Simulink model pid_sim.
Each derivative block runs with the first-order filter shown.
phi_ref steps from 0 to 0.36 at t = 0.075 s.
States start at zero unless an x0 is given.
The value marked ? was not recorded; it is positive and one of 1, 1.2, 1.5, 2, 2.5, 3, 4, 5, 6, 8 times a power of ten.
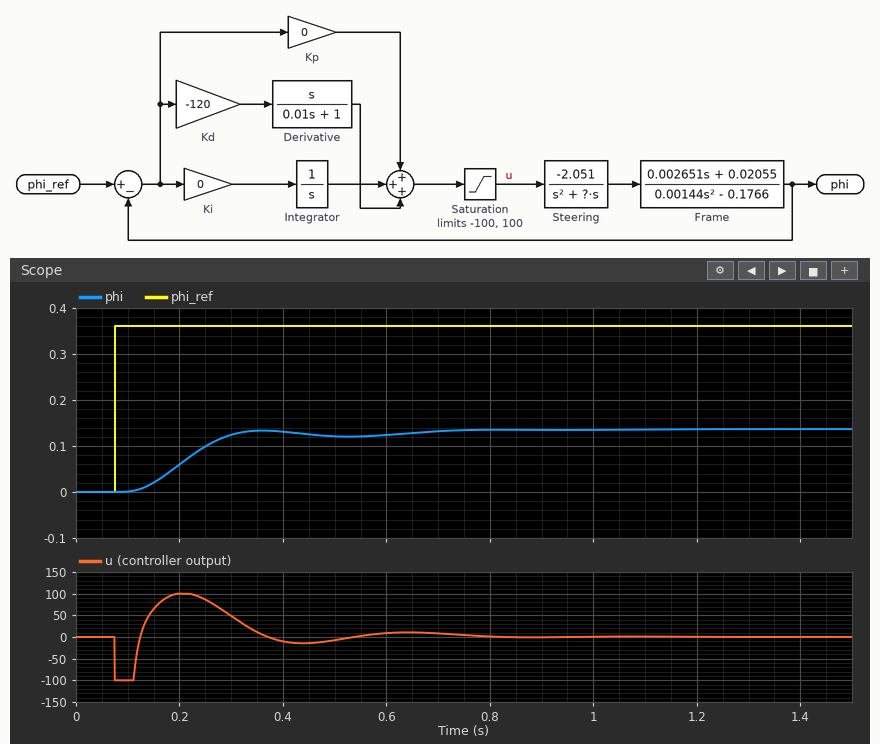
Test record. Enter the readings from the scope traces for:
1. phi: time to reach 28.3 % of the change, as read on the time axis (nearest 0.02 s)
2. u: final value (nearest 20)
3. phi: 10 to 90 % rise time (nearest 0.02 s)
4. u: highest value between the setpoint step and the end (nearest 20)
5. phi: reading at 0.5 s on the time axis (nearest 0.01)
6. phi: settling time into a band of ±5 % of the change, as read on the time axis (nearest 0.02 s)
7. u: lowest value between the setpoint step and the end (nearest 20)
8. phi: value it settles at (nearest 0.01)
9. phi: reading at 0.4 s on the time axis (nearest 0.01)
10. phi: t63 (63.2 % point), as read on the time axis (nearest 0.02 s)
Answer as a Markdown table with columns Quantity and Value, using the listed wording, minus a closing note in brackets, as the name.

| Quantity | Value |
|---|---|
| phi: time to reach 28.3 % of the change, as read on the time axis | 0.18 s |
| u: final value | 0 |
| phi: 10 to 90 % rise time | 0.16 s |
| u: highest value between the setpoint step and the end | 100 |
| phi: reading at 0.5 s on the time axis | 0.12 |
| phi: settling time into a band of ±5 % of the change, as read on the time axis | 0.68 s |
| u: lowest value between the setpoint step and the end | -100 |
| phi: value it settles at | 0.14 |
| phi: reading at 0.4 s on the time axis | 0.13 |
| phi: t63 (63.2 % point), as read on the time axis | 0.24 s |
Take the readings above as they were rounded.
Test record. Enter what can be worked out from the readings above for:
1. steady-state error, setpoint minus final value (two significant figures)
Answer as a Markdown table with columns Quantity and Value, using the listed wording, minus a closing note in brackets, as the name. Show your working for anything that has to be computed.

| Quantity | Value |
|---|---|
| steady-state error, setpoint minus final value | 0.36 - 0.14 = 0.22 |
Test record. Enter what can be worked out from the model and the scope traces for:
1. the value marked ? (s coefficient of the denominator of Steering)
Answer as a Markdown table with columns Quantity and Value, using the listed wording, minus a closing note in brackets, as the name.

| Quantity | Value |
|---|---|
| the value marked ? | 20 |
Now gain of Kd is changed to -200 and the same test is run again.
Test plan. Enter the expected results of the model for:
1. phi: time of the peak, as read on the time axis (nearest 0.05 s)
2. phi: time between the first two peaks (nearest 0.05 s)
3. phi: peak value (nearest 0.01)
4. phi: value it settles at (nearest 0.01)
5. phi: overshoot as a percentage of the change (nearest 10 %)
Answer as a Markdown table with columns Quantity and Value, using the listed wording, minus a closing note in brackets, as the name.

| Quantity | Value |
|---|---|
| phi: time of the peak, as read on the time axis | 0.30 s |
| phi: time between the first two peaks | 0.30 s |
| phi: peak value | 0.09 |
| phi: value it settles at | 0.08 |
| phi: overshoot as a percentage of the change | 20 % |
